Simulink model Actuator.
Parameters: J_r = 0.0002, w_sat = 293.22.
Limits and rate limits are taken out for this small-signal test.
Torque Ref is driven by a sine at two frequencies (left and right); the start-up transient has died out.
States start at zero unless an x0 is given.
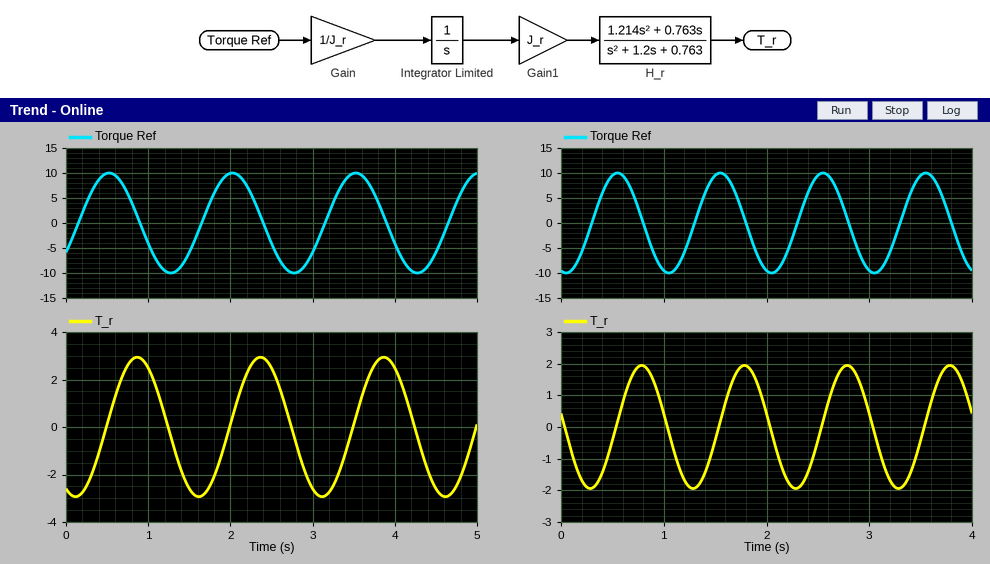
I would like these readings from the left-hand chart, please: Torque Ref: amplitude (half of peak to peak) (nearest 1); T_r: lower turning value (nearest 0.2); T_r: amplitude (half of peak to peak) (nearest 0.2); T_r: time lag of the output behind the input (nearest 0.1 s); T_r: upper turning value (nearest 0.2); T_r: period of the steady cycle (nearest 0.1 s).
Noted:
10
-3.0
3.0
0.3 s
3.0
1.5 s
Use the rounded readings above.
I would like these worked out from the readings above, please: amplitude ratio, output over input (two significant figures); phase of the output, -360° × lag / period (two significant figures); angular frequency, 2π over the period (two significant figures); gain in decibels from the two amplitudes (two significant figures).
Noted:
0.30
-72°
4.2 rad/s
-10 dB
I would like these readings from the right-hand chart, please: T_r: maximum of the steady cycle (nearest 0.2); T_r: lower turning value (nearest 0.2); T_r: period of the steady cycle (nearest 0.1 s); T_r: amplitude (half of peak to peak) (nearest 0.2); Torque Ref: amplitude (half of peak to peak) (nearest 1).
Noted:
2.0
-2.0
1.0 s
2.0
10
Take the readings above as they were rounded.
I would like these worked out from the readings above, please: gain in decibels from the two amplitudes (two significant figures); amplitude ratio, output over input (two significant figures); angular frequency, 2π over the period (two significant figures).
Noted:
-14 dB
0.20
6.3 rad/s
